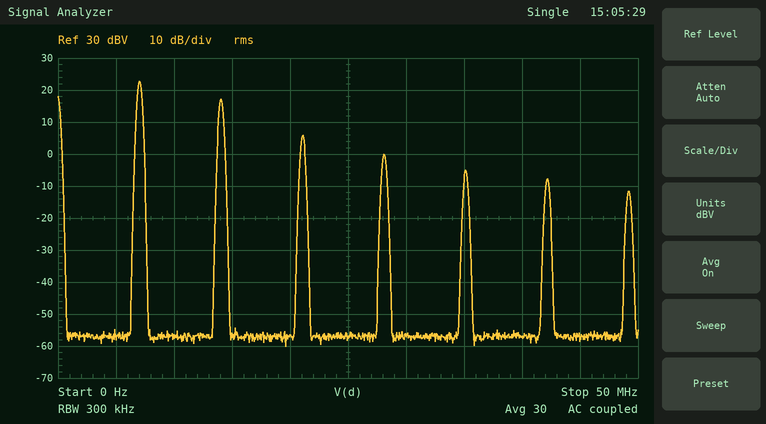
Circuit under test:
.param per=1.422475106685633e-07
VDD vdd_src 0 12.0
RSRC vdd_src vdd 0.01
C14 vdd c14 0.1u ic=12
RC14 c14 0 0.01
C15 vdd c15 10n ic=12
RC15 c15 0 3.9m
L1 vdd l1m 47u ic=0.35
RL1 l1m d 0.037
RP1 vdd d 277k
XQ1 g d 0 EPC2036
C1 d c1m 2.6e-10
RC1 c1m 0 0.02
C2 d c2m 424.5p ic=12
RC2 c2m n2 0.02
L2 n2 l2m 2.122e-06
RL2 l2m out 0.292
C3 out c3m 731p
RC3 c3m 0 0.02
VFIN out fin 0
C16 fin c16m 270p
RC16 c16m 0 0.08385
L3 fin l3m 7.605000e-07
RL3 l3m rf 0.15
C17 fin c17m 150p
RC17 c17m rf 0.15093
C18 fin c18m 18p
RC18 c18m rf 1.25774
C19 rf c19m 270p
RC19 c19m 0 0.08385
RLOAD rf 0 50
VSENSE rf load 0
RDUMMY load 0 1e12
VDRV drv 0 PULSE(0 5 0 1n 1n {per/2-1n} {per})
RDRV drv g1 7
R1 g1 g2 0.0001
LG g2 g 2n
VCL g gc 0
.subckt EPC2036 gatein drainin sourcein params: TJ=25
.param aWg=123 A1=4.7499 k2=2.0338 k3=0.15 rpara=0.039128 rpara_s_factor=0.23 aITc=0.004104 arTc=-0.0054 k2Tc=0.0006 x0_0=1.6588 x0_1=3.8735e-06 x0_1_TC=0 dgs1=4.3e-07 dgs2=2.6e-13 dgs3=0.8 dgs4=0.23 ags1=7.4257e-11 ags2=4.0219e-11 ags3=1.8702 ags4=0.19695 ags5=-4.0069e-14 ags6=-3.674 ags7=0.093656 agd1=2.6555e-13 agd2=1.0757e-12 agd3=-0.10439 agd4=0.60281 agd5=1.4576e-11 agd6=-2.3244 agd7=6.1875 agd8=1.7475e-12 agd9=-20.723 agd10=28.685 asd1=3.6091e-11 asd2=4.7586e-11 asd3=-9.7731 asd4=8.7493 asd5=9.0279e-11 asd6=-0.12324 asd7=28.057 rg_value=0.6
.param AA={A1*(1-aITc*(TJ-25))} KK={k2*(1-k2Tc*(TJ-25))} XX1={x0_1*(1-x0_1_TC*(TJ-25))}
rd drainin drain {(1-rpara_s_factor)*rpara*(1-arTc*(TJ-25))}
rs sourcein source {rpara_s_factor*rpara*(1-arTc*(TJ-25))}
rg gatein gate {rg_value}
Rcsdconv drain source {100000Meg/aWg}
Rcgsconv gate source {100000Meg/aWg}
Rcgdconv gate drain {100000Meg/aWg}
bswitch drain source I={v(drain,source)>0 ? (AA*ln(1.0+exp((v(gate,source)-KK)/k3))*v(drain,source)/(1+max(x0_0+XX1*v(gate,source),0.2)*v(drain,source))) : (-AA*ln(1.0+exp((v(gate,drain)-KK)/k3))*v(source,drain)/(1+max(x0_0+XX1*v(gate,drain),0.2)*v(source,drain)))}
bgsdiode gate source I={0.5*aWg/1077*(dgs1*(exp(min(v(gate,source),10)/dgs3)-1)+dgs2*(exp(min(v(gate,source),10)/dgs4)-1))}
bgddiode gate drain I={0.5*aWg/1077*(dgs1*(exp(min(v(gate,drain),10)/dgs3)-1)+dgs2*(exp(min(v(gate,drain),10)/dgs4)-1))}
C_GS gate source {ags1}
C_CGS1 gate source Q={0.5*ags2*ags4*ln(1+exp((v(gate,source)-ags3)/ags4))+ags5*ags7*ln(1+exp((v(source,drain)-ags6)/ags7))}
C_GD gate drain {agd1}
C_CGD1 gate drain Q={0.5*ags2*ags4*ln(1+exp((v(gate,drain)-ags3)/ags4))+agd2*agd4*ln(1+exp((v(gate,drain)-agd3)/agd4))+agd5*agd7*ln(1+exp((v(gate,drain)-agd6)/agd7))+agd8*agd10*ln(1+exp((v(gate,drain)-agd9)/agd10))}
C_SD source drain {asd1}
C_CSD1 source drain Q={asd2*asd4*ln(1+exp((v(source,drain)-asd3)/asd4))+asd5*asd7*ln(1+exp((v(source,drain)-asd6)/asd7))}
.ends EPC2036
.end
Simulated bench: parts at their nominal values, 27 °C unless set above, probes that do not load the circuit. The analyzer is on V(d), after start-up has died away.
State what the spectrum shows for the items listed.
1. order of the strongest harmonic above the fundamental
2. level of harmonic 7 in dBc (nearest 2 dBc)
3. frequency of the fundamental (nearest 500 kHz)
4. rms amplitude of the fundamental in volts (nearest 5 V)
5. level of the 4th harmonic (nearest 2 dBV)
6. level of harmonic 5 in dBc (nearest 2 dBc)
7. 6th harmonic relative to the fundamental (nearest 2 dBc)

2
-34 dBc
7.0 MHz
15 V
0 dBV
-28 dBc
-30 dBc
